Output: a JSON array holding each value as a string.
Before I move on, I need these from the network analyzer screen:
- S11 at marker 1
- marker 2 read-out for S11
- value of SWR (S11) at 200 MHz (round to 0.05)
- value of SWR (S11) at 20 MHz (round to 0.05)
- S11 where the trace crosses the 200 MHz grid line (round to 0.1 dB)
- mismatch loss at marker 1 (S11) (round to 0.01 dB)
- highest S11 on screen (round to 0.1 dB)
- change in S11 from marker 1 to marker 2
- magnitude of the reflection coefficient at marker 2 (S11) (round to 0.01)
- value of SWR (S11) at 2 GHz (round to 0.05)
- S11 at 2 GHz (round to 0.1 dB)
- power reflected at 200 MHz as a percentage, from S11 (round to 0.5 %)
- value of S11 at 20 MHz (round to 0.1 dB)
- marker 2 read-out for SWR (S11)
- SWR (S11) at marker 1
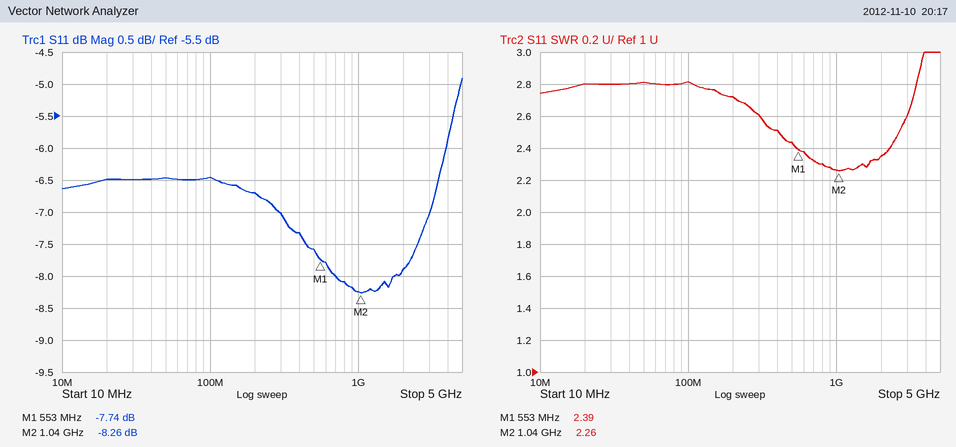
["-7.74 dB", "-8.26 dB", "2.70", "2.80", "-6.7 dB", "0.80 dB", "-4.9 dB", "-0.52 dB", "0.39", "2.35", "-7.9 dB", "21.5 %", "-6.5 dB", "2.26", "2.39"]
